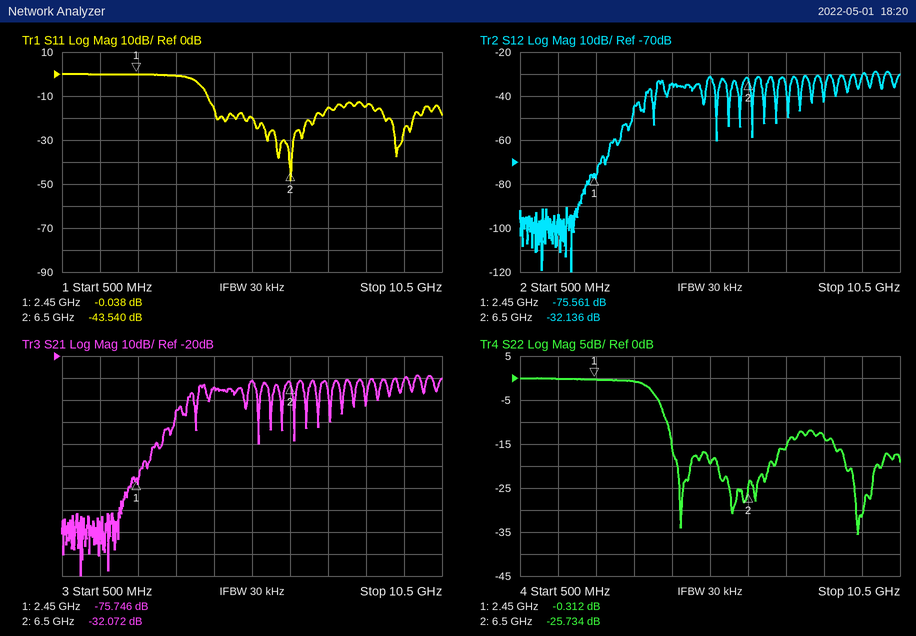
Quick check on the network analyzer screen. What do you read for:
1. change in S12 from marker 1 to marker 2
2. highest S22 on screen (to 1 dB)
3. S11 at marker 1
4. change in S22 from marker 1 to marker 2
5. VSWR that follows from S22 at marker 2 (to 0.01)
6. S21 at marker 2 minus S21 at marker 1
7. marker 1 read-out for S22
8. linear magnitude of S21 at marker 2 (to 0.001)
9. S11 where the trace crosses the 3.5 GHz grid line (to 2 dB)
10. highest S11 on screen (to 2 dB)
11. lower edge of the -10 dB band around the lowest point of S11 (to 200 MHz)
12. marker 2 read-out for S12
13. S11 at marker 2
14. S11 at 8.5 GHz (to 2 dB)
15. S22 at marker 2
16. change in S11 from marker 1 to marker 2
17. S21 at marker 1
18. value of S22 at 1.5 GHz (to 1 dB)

43.425 dB
0 dB
-0.038 dB
-25.422 dB
1.11
43.674 dB
-0.312 dB
0.025
0 dB
0 dB
4.4 GHz
-32.136 dB
-43.540 dB
-14 dB
-25.734 dB
-43.502 dB
-75.746 dB
0 dB
